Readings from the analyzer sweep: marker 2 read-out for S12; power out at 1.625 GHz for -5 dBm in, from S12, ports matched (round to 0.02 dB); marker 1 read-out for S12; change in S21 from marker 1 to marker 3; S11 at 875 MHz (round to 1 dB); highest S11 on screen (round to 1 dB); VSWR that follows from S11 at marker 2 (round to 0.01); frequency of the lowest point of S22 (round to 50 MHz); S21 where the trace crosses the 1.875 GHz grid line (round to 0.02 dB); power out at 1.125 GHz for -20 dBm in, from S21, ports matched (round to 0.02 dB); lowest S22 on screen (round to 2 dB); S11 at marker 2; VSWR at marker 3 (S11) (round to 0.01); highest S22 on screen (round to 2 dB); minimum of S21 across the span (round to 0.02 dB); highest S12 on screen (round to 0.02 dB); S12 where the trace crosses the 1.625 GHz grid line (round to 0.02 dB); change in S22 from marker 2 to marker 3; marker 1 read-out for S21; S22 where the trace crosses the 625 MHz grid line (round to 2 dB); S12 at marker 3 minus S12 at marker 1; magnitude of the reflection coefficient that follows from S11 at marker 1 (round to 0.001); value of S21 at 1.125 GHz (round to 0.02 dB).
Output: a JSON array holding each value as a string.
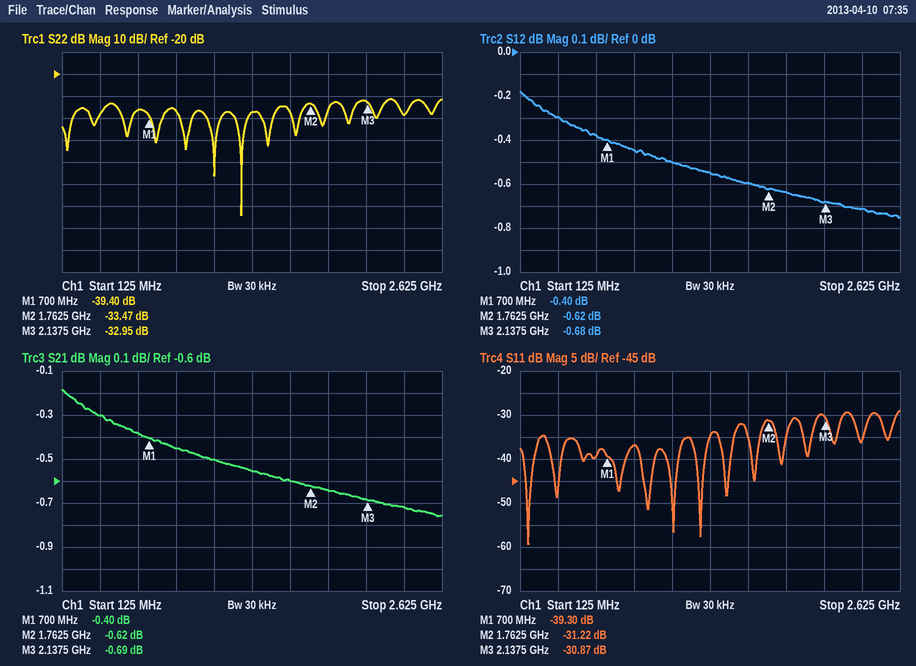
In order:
["-0.62 dB", "-5.60 dBm", "-0.40 dB", "-0.29 dB", "-37 dB", "-29 dB", "1.06", "1.30 GHz", "-0.64 dB", "-20.50 dBm", "-84 dB", "-31.22 dB", "1.06", "-32 dB", "-0.76 dB", "-0.18 dB", "-0.60 dB", "0.52 dB", "-0.40 dB", "-36 dB", "-0.28 dB", "0.011", "-0.50 dB"]
